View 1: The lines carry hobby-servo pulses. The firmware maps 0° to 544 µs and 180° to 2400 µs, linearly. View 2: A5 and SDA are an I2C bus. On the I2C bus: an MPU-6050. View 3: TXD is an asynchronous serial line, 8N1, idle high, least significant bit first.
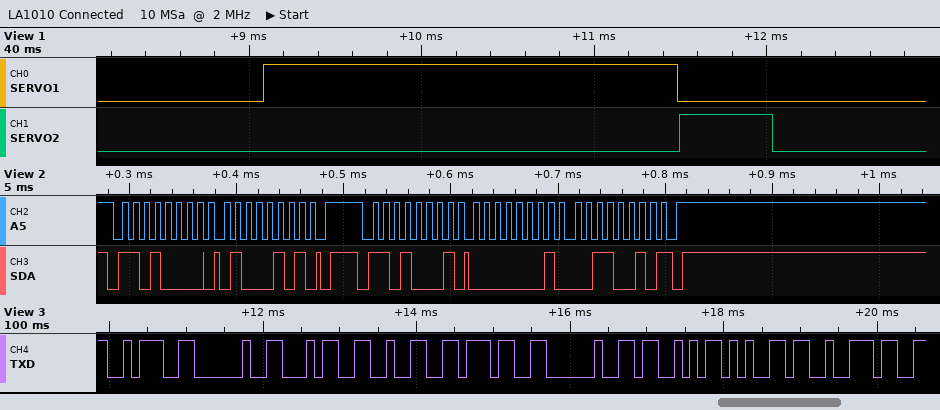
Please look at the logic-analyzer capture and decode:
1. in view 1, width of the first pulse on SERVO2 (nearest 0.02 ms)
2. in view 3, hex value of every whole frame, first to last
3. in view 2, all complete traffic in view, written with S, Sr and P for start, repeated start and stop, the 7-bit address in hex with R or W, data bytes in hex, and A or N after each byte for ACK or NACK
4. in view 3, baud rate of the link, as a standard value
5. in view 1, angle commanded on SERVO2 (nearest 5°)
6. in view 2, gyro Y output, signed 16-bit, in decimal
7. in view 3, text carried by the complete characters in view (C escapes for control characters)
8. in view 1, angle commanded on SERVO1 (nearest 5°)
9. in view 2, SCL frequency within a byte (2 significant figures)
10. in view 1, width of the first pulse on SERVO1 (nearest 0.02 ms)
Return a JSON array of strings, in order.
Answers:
["0.54 ms", "3A 20 34 32 37 20 53 65 72", "S 68W A 45 A P S 68R A 01 A 32 N P", "9600 baud", "0°", "306", "\": 427 Ser\"", "180°", "100 kHz", "2.40 ms"]
